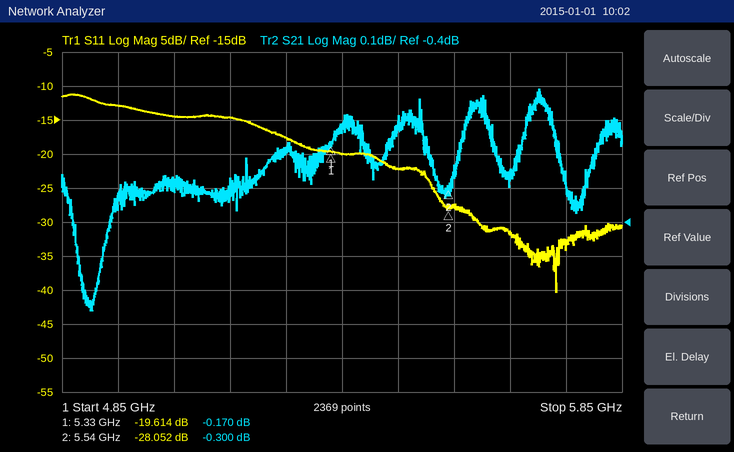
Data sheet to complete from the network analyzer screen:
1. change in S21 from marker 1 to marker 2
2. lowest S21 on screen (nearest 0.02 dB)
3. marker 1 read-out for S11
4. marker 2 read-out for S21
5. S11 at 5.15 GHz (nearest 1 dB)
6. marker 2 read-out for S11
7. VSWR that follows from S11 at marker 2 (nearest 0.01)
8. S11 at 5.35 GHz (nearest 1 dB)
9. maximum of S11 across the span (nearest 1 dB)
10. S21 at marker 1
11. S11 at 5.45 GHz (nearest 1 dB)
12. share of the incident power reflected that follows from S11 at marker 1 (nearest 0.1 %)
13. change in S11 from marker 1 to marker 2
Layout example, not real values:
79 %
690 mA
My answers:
-0.130 dB
-0.66 dB
-19.614 dB
-0.300 dB
-15 dB
-28.052 dB
1.08
-20 dB
-11 dB
-0.170 dB
-22 dB
1.1 %
-8.438 dB
